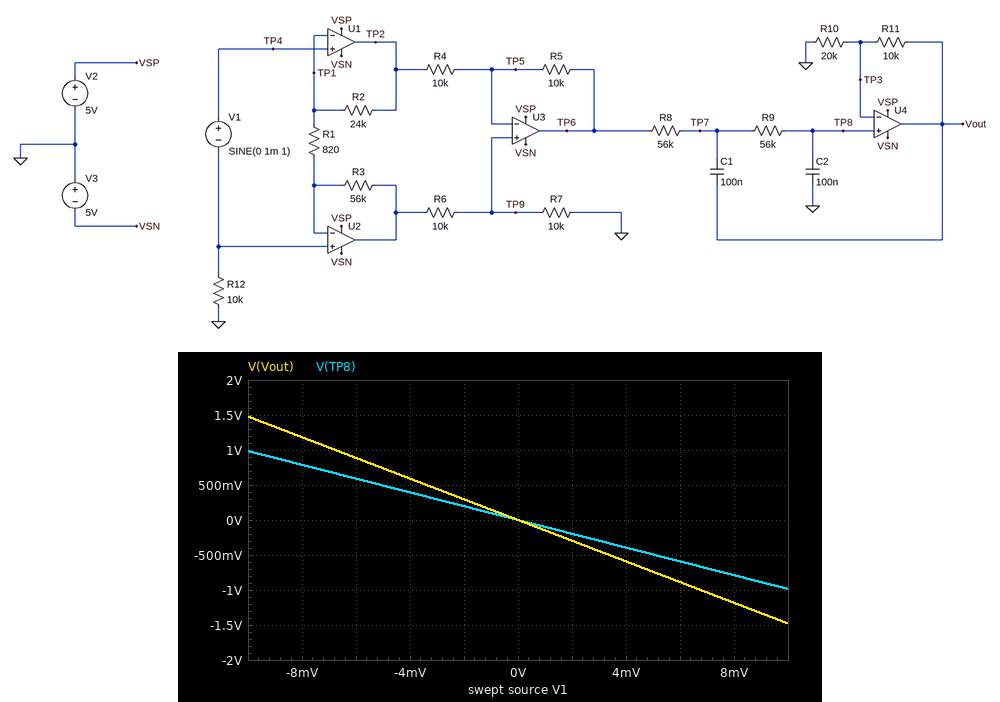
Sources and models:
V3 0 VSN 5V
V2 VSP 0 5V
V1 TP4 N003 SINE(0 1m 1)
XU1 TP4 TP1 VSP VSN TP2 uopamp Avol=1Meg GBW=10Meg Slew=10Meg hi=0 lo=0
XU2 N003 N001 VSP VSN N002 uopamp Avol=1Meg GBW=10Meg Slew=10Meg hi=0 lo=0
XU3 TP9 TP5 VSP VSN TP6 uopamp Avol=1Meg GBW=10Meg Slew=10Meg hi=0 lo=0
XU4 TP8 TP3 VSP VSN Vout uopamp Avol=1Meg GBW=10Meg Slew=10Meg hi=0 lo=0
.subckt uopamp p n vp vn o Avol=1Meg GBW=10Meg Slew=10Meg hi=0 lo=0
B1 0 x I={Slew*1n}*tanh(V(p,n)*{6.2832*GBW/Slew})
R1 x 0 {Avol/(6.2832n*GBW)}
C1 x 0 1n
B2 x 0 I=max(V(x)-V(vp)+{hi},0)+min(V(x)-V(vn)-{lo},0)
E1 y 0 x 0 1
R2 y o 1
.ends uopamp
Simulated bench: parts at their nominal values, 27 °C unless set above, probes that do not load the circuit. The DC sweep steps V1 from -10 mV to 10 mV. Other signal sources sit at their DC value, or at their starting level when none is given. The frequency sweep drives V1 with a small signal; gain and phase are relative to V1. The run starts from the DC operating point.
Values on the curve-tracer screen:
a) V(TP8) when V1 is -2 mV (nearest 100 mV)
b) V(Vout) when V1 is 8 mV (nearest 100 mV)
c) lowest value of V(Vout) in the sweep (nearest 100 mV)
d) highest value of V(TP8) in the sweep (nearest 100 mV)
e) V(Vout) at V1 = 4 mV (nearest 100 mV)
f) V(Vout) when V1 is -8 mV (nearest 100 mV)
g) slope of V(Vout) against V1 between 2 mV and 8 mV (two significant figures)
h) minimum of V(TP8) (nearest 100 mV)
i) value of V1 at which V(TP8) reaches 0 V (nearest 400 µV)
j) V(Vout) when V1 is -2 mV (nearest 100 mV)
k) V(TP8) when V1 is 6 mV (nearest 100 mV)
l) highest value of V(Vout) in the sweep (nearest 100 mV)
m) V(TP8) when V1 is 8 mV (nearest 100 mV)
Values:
200 mV
-1.2 V
-1.5 V
1.0 V
-600 mV
1.2 V
-150 V/V
-1.0 V
0 V
300 mV
-600 mV
1.5 V
-800 mV
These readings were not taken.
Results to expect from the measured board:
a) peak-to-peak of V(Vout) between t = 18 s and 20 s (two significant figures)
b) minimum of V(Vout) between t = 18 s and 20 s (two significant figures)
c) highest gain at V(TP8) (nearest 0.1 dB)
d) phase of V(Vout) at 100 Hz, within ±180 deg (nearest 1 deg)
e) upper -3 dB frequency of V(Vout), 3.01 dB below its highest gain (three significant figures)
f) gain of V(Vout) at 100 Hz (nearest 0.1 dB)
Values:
300 mV
-150 mV
39.9 dB
25 deg
26.7 Hz
21.4 dB
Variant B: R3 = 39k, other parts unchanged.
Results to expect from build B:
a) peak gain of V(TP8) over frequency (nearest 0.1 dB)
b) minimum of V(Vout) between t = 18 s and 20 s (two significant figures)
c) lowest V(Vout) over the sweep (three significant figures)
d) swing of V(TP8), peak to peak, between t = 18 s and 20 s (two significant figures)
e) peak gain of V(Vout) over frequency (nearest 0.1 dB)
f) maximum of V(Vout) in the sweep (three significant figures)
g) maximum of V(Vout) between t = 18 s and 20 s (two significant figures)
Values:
37.8 dB
-120 mV
-1.17 V
160 mV
41.3 dB
1.17 V
120 mV
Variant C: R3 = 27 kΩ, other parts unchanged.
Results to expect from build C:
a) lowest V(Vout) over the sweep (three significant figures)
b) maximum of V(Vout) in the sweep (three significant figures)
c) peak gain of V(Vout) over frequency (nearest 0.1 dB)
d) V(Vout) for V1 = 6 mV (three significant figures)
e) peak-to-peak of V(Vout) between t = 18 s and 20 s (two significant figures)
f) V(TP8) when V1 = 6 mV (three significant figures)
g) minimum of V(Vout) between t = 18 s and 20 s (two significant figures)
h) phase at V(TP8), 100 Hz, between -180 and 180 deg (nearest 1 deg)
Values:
-948 mV
948 mV
39.5 dB
-569 mV
190 mV
-379 mV
-95 mV
25 deg
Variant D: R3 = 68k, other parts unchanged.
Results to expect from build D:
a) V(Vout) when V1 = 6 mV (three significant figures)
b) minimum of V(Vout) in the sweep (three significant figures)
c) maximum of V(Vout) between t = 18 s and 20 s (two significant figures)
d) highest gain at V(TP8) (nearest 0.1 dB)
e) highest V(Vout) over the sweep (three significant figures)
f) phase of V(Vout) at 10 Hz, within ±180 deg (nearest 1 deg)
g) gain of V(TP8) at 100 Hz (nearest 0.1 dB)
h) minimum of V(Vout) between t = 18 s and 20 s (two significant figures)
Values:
-1.02 V
-1.70 V
170 mV
41.1 dB
1.70 V
149 deg
19.1 dB
-170 mV
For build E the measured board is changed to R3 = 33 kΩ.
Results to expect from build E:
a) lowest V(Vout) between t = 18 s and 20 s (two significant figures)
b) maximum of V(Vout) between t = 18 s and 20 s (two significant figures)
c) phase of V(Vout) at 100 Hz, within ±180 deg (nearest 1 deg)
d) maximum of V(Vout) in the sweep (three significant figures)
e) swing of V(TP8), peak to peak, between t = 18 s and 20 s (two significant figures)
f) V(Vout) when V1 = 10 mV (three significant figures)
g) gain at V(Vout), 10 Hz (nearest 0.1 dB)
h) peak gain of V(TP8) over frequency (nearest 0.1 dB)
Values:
-110 mV
110 mV
25 deg
1.06 V
140 mV
-1.06 V
40.3 dB
37.0 dB
